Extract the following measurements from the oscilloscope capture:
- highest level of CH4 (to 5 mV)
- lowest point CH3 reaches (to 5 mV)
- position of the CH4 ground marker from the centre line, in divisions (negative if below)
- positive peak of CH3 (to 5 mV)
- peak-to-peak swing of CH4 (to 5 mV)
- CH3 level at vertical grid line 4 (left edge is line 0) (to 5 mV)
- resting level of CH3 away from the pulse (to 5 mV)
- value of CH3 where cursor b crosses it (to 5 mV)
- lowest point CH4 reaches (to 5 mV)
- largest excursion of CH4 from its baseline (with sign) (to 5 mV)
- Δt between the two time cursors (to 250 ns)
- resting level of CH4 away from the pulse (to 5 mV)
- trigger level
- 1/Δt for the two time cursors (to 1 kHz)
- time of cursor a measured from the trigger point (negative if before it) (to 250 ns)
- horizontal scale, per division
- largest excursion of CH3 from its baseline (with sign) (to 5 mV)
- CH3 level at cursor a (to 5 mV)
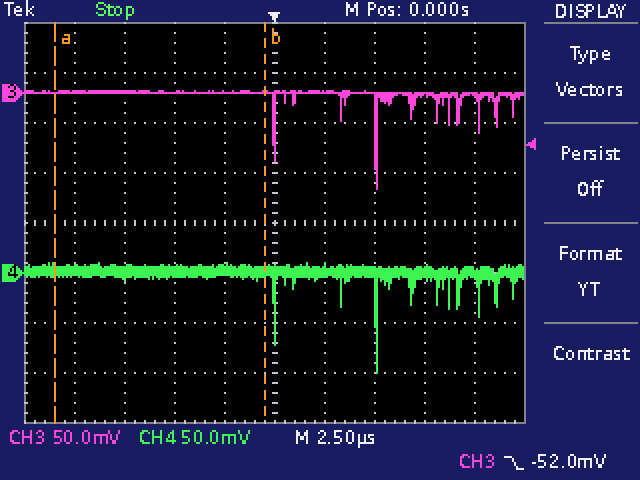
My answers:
10 mV
-95 mV
-1.0 div
0 mV
110 mV
0 mV
0 mV
0 mV
-100 mV
-100 mV
10.50 µs
0 mV
-52.0 mV
95 kHz
-11.00 µs
2.5 µs
-95 mV
0 mV
